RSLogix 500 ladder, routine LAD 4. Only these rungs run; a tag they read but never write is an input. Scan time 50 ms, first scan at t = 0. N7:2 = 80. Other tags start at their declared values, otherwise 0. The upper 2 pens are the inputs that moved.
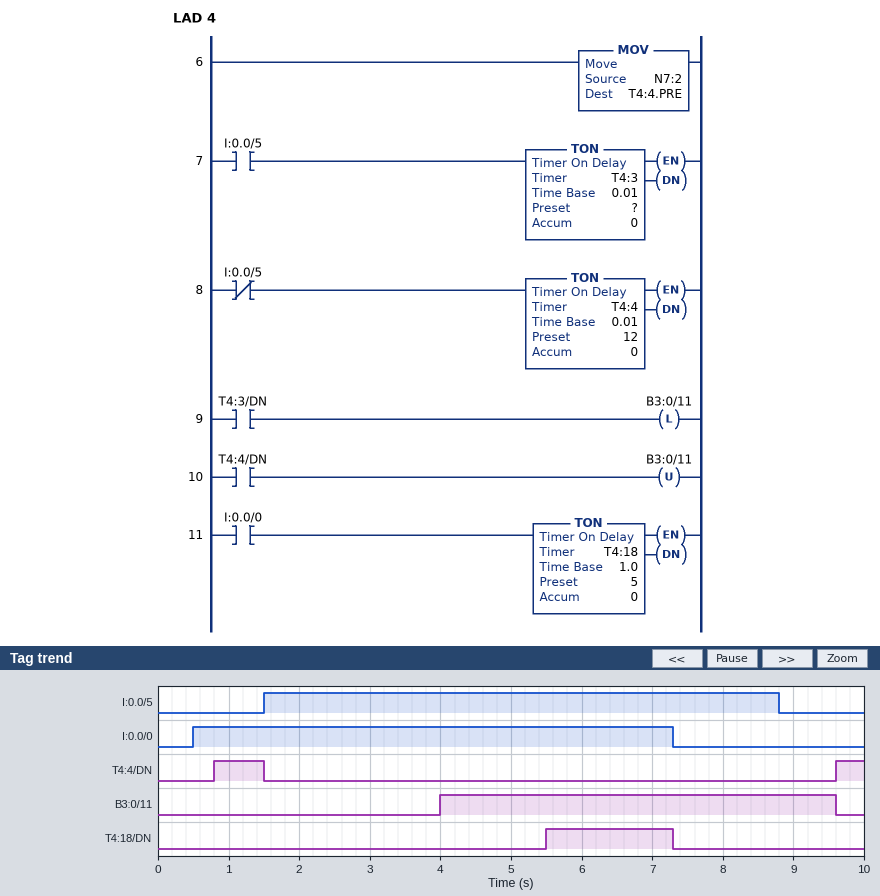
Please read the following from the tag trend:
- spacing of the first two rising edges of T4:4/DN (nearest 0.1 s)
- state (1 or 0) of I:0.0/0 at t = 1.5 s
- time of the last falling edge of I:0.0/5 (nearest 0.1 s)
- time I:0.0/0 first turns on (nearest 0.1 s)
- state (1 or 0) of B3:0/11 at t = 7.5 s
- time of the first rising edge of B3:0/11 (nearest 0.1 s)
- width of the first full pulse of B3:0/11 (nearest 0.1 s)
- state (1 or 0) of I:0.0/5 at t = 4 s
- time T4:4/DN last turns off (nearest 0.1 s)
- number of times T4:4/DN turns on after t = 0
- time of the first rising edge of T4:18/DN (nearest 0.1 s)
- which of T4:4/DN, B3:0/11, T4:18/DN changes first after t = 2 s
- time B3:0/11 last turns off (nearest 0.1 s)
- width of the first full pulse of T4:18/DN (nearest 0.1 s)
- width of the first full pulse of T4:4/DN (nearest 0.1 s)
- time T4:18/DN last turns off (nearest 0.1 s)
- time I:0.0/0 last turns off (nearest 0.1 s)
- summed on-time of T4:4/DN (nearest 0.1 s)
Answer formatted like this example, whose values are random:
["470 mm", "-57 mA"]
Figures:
["8.8 s", "1", "8.8 s", "0.5 s", "1", "4.0 s", "5.6 s", "1", "1.5 s", "2", "5.5 s", "B3:0/11", "9.6 s", "1.8 s", "0.7 s", "7.3 s", "7.3 s", "1.1 s"]
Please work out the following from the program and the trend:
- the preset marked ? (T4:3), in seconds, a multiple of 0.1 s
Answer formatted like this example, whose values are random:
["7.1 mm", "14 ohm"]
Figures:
["2.5 s"]
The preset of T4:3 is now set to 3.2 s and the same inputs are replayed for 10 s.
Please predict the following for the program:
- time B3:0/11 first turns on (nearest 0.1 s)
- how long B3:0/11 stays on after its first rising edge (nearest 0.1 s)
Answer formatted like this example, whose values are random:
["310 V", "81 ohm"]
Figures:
["4.7 s", "4.9 s"]
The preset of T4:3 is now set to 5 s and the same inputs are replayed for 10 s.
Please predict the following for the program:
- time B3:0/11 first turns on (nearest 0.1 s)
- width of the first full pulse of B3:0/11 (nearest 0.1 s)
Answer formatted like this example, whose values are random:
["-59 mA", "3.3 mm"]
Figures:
["6.5 s", "3.1 s"]
